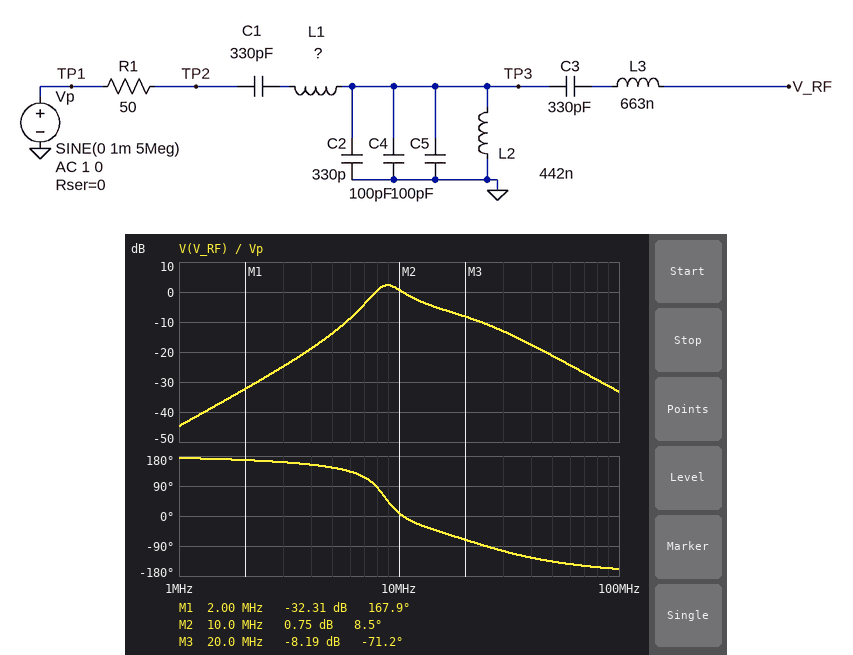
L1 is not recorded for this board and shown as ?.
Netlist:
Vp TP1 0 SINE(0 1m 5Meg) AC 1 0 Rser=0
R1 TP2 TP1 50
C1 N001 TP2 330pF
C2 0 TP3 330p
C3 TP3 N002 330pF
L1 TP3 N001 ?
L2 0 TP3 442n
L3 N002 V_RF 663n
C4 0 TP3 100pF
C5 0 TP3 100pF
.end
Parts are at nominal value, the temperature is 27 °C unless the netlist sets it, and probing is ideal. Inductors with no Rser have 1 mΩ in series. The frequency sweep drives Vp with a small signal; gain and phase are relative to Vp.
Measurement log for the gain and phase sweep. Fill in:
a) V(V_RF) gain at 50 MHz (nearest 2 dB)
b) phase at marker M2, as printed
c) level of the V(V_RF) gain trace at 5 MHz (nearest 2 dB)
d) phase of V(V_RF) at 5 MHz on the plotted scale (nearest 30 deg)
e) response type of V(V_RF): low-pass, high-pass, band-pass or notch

-22 dB
8.5 deg
-14 dB
150 deg
band-pass
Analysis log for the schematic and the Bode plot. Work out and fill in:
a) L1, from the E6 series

220 nH
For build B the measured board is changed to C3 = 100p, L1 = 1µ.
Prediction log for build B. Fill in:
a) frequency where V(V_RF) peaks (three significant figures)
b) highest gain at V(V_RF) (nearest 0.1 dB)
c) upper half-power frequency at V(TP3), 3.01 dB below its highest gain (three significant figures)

12.4 MHz
1.9 dB
14.3 MHz
